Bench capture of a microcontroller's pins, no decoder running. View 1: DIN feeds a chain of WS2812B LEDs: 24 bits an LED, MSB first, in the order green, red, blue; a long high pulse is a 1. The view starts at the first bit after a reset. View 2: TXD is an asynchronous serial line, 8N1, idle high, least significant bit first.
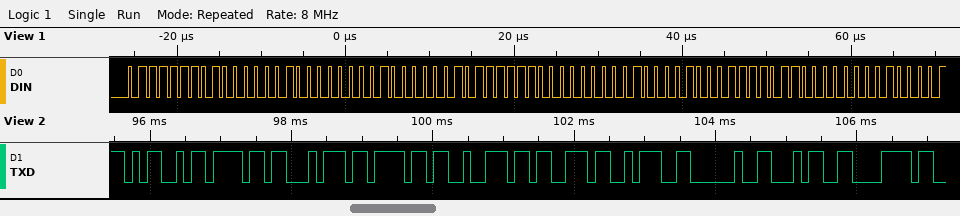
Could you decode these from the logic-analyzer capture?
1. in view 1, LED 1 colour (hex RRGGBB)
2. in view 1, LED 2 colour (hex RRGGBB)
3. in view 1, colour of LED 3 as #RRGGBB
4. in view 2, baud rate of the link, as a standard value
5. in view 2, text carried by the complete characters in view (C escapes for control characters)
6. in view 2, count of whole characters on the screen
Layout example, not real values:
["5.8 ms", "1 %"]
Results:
["#817E00", "#7E8100", "#7B8400", "9600 baud", "\"Motors: 4x\"", "10"]
